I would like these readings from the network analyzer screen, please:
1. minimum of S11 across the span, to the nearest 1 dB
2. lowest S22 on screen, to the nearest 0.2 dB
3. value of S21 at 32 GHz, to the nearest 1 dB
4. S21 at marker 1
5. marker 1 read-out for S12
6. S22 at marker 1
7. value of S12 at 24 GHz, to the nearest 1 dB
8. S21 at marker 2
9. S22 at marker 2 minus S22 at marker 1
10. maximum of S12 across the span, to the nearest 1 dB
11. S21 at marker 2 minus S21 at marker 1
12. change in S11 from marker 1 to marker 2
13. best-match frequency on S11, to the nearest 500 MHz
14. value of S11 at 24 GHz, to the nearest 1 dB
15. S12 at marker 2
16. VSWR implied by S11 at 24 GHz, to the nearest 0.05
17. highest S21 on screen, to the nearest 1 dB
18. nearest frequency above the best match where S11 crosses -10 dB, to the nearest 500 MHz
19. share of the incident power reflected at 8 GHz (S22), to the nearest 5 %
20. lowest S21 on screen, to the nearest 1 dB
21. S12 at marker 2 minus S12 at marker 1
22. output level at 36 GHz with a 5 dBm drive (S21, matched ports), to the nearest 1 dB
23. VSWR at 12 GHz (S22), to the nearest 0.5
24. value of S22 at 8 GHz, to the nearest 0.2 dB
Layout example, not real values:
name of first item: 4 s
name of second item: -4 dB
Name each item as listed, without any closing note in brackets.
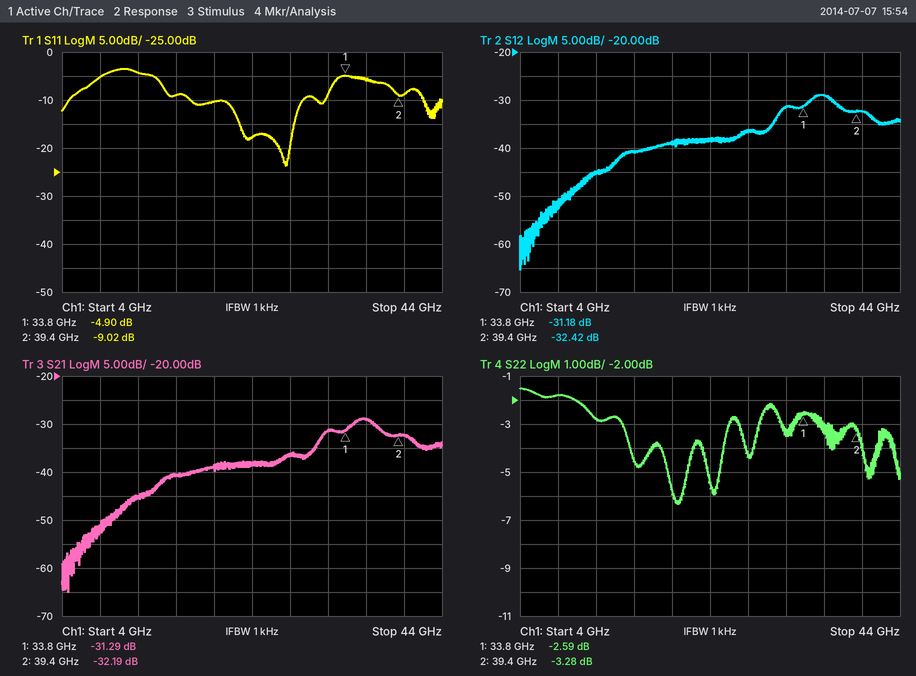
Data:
minimum of S11 across the span, to the nearest 1 dB: -24 dB
lowest S22 on screen, to the nearest 0.2 dB: -6.4 dB
value of S21 at 32 GHz, to the nearest 1 dB: -31 dB
S21 at marker 1: -31.29 dB
marker 1 read-out for S12: -31.18 dB
S22 at marker 1: -2.59 dB
value of S12 at 24 GHz, to the nearest 1 dB: -38 dB
S21 at marker 2: -32.19 dB
S22 at marker 2 minus S22 at marker 1: -0.69 dB
maximum of S12 across the span, to the nearest 1 dB: -29 dB
S21 at marker 2 minus S21 at marker 1: -0.90 dB
change in S11 from marker 1 to marker 2: -4.12 dB
best-match frequency on S11, to the nearest 500 MHz: 27.5 GHz
value of S11 at 24 GHz, to the nearest 1 dB: -18 dB
S12 at marker 2: -32.42 dB
VSWR implied by S11 at 24 GHz, to the nearest 0.05: 1.30
highest S21 on screen, to the nearest 1 dB: -29 dB
nearest frequency above the best match where S11 crosses -10 dB, to the nearest 500 MHz: 29.5 GHz
share of the incident power reflected at 8 GHz (S22), to the nearest 5 %: 65 %
lowest S21 on screen, to the nearest 1 dB: -65 dB
S12 at marker 2 minus S12 at marker 1: -1.24 dB
output level at 36 GHz with a 5 dBm drive (S21, matched ports), to the nearest 1 dB: -24 dBm
VSWR at 12 GHz (S22), to the nearest 0.5: 6.5
value of S22 at 8 GHz, to the nearest 0.2 dB: -1.8 dB
